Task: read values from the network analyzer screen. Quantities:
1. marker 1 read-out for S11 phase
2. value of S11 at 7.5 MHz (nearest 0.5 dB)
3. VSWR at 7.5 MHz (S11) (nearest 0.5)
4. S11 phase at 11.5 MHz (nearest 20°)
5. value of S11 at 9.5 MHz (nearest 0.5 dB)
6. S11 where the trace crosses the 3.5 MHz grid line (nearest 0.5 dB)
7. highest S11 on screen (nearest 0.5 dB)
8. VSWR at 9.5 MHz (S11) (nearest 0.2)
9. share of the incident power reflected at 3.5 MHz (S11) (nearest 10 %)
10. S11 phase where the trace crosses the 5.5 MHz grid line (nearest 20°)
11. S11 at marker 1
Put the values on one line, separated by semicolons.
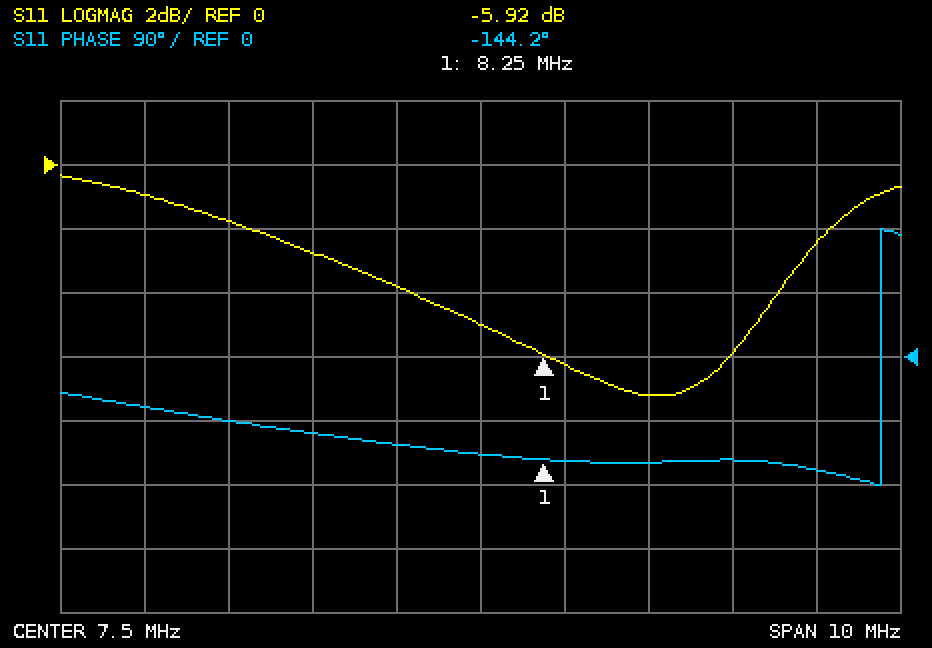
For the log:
-144.2°; -5.0 dB; 3.5; -160°; -7.0 dB; -1.0 dB; -0.5 dB; 2.6; 80 %; -100°; -5.92 dB
